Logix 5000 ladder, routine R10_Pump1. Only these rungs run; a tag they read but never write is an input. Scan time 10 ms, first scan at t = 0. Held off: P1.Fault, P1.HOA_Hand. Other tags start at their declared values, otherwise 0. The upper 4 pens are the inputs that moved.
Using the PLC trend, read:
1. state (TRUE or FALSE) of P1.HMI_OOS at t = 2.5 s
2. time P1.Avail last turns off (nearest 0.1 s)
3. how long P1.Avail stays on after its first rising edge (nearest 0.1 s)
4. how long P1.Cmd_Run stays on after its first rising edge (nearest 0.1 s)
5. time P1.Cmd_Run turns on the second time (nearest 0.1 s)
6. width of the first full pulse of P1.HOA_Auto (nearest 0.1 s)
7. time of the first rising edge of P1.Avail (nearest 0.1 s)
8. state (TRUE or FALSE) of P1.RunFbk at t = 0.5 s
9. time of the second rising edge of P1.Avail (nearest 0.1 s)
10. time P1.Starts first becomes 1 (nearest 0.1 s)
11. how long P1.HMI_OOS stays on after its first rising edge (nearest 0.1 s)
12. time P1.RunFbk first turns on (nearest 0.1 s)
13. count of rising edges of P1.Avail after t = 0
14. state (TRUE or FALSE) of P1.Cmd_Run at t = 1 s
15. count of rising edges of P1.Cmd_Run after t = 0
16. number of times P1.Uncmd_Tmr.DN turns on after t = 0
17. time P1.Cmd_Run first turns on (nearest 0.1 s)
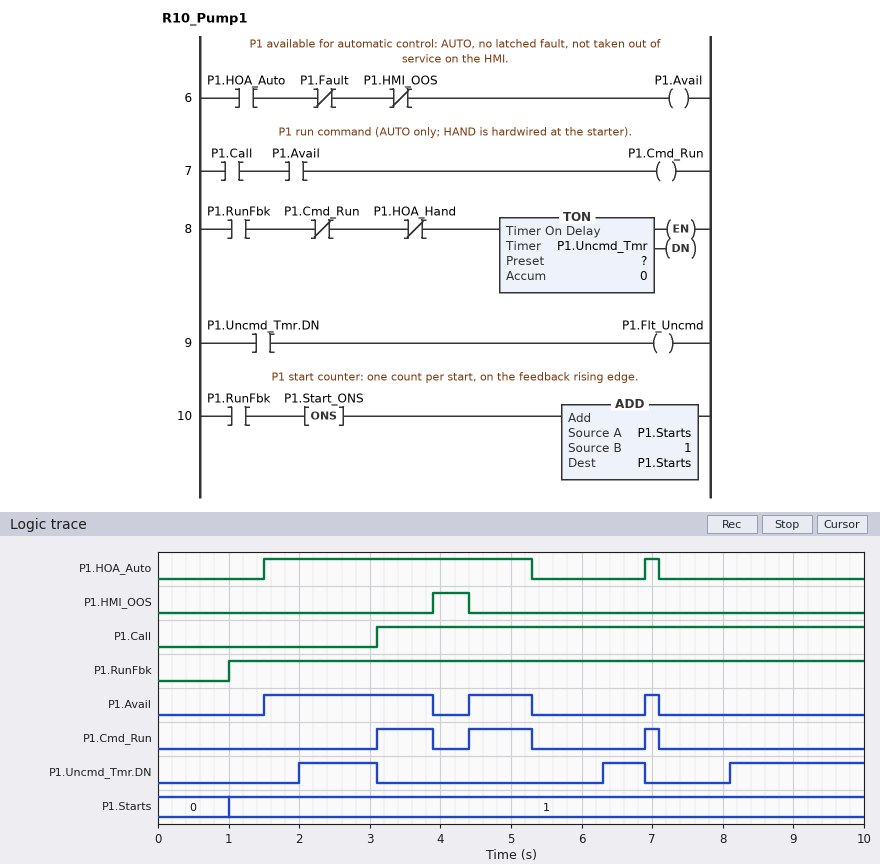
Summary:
FALSE
7.1 s
2.4 s
0.8 s
4.4 s
3.8 s
1.5 s
FALSE
4.4 s
1.0 s
0.5 s
1.0 s
3
FALSE
3
3
3.1 s
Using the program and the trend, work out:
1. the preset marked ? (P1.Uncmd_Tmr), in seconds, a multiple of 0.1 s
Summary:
1.0 s
